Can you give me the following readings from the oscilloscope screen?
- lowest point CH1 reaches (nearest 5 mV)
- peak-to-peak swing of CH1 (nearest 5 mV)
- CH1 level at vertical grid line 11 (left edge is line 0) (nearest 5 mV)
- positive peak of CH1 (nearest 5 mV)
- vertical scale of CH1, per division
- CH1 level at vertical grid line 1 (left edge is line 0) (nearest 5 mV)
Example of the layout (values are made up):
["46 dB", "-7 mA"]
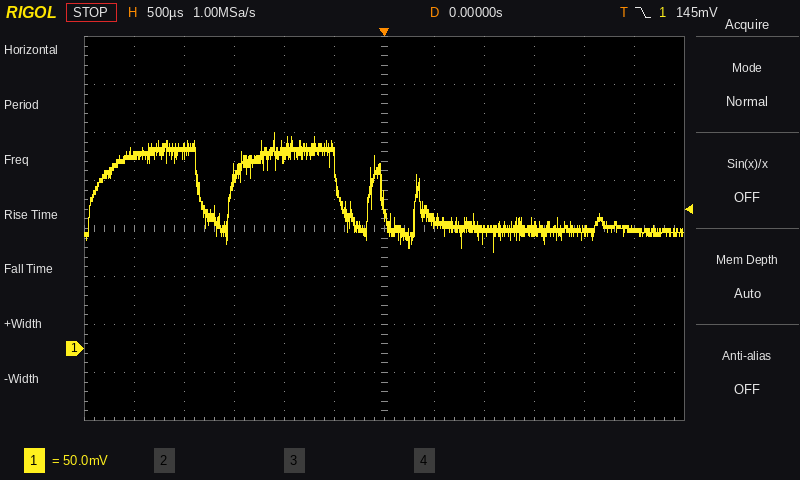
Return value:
["100 mV", "125 mV", "125 mV", "225 mV", "50 mV", "200 mV"]
